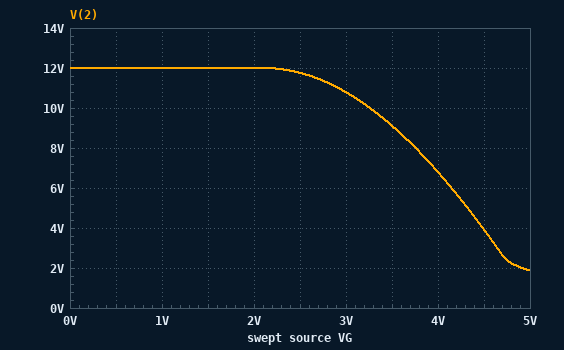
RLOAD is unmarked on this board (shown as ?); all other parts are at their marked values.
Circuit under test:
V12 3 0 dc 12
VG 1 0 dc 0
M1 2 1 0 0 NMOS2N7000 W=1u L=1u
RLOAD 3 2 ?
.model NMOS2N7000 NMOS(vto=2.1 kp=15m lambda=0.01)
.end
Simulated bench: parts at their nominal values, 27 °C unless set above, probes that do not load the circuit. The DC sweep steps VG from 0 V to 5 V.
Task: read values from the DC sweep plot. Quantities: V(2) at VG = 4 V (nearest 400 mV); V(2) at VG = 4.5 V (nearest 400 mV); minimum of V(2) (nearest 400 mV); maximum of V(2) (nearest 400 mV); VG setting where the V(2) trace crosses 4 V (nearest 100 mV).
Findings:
6.8 V
4.0 V
2.0 V
12.0 V
4.5 V
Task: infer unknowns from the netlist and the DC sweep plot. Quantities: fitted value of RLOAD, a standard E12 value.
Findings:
180 Ω
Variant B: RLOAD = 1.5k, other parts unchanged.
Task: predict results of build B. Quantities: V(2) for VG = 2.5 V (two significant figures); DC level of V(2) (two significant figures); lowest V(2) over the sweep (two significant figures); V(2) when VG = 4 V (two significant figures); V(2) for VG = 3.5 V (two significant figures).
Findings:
10 V
12 V
190 mV
300 mV
430 mV
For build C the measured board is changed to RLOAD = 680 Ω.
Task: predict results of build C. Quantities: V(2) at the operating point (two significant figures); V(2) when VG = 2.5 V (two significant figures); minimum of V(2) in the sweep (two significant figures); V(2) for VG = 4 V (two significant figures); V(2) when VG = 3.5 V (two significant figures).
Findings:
12 V
11 V
420 mV
710 mV
1.8 V
